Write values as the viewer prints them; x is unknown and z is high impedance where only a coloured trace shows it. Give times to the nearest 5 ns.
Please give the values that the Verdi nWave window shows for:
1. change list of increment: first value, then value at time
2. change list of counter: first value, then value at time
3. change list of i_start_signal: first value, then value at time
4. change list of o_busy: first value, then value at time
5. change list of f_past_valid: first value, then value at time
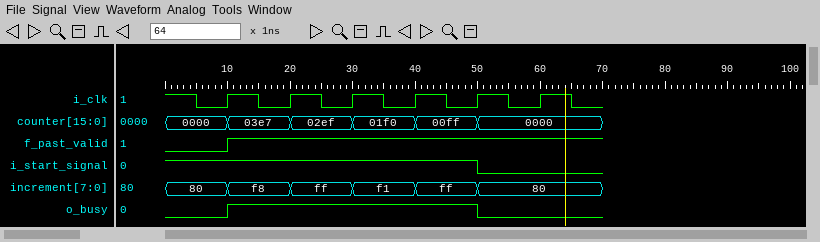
80, f8 at 10 ns, ff at 20 ns, f1 at 30 ns, ff at 40 ns, 80 at 50 ns
0000, 03e7 at 10 ns, 02ef at 20 ns, 01f0 at 30 ns, 00ff at 40 ns, 0000 at 50 ns
1, 0 at 50 ns
0, 1 at 10 ns, 0 at 50 ns
0, 1 at 10 ns
